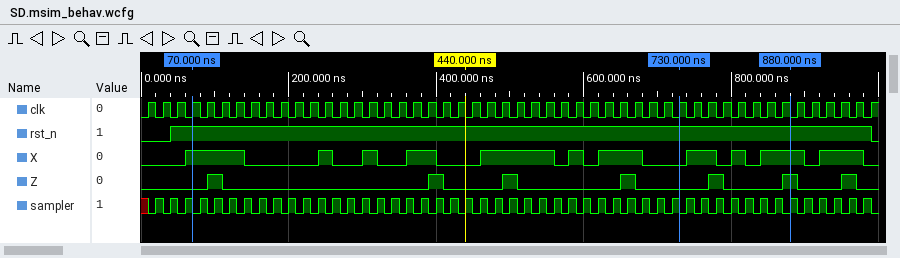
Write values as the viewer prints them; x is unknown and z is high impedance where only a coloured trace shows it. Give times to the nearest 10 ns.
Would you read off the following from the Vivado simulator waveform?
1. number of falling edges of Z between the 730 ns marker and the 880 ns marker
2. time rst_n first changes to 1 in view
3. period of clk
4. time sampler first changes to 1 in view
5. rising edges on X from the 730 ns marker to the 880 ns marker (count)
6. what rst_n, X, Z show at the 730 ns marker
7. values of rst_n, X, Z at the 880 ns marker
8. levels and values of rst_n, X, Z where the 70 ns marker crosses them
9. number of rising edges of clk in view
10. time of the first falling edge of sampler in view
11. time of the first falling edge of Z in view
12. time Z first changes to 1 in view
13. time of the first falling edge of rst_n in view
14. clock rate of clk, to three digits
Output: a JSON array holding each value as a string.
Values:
["1", "40 ns", "20 ns", "20 ns", "3", "rst_n=1, X=0, Z=0", "rst_n=1, X=1, Z=1", "rst_n=1, X=1, Z=0", "50", "30 ns", "110 ns", "90 ns", "990 ns", "50.0 MHz"]
